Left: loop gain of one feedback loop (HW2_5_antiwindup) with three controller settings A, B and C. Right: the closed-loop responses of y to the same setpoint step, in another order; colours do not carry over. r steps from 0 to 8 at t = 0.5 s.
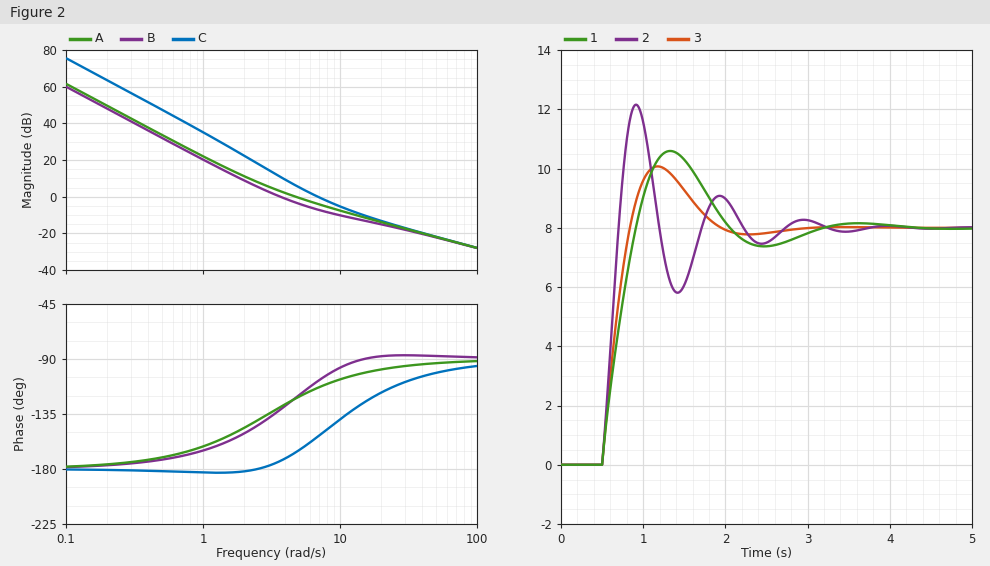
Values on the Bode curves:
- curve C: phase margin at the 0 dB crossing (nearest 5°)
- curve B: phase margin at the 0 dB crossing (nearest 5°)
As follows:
25°
50°
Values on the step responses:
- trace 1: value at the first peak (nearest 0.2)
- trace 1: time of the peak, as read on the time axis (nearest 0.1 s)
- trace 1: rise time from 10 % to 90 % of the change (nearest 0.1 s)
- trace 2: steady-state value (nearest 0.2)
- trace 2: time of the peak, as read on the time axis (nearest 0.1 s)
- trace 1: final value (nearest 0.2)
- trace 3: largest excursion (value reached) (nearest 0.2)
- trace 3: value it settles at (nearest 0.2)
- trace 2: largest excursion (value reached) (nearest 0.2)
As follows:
10.6
1.3 s
0.3 s
8.0
0.9 s
8.0
10.0
8.0
12.2
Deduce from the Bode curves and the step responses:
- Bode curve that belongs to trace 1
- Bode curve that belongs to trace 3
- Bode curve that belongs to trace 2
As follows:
B
A
C
